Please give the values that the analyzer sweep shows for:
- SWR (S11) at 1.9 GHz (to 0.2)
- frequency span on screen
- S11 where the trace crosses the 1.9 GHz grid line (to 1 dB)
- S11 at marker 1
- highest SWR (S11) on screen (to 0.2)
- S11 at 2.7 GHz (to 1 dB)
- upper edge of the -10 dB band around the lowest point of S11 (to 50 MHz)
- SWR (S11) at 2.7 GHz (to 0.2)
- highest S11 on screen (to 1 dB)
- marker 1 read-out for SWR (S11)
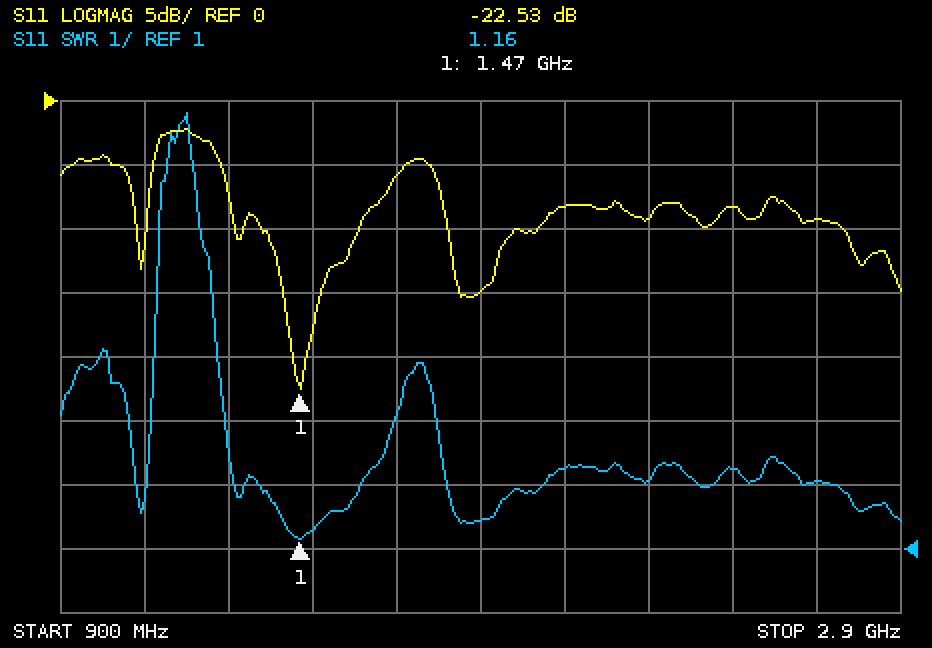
1.4
2 GHz
-15 dB
-22.53 dB
7.8
-9 dB
1.60 GHz
2.0
-2 dB
1.16
